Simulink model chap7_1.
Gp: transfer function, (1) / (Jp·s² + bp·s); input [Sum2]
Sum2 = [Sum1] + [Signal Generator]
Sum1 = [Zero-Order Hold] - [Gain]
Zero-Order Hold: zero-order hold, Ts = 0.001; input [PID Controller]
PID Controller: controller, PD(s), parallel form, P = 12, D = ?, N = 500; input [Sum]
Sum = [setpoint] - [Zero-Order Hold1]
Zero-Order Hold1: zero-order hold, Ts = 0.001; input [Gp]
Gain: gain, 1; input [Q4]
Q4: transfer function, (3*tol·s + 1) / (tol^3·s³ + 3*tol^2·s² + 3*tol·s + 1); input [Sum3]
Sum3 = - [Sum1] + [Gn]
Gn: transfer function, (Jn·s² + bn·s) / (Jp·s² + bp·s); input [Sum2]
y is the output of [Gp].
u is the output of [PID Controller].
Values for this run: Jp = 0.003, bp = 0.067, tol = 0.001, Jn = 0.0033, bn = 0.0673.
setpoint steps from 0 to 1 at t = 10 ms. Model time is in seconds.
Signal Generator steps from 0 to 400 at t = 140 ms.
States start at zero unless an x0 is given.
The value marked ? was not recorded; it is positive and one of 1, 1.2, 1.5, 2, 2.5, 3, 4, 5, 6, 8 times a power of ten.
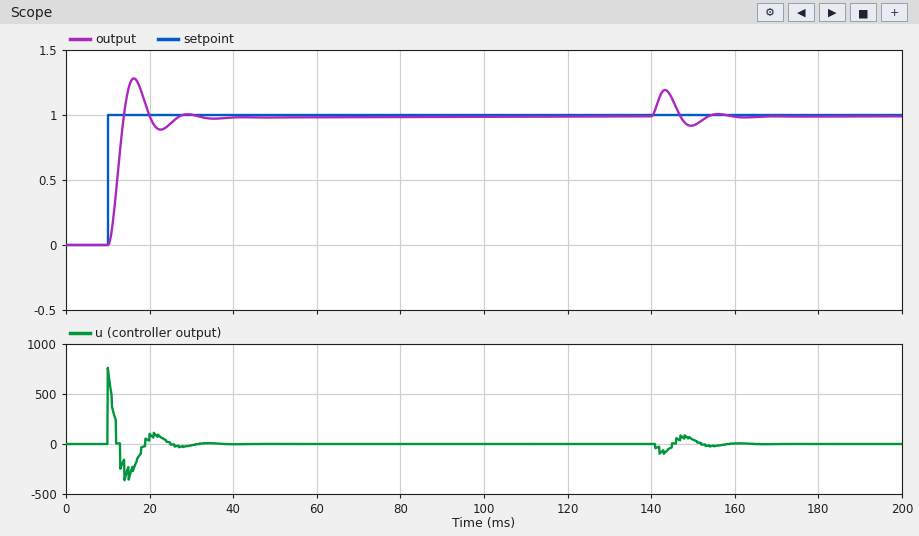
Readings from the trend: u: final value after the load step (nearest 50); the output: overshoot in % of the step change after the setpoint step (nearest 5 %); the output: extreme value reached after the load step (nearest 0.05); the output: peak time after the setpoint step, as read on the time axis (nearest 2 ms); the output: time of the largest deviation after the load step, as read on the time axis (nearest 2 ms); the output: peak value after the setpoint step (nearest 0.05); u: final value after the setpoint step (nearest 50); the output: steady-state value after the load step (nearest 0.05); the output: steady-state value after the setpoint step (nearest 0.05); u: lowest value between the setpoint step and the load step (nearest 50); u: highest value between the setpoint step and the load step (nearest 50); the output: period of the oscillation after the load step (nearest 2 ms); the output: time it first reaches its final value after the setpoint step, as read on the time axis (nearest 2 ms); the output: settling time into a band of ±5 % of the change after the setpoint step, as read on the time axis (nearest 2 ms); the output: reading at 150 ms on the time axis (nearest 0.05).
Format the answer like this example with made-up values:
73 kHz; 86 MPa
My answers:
0; 30 %; 1.20; 16 ms; 144 ms; 1.30; 0; 1.00; 1.00; -350; 750; 12 ms; 14 ms; 26 ms; 0.90
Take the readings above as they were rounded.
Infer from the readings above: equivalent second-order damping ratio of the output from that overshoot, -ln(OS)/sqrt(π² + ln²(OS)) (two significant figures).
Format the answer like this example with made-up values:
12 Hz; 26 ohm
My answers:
0.36
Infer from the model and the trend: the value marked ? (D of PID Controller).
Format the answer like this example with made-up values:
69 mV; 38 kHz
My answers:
1.5
